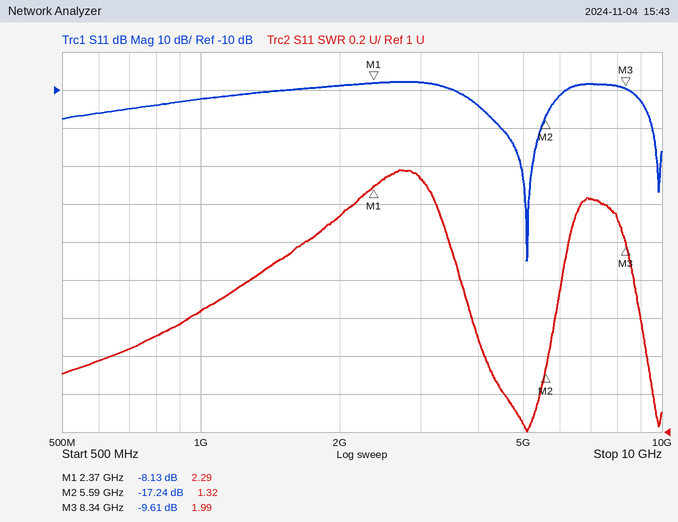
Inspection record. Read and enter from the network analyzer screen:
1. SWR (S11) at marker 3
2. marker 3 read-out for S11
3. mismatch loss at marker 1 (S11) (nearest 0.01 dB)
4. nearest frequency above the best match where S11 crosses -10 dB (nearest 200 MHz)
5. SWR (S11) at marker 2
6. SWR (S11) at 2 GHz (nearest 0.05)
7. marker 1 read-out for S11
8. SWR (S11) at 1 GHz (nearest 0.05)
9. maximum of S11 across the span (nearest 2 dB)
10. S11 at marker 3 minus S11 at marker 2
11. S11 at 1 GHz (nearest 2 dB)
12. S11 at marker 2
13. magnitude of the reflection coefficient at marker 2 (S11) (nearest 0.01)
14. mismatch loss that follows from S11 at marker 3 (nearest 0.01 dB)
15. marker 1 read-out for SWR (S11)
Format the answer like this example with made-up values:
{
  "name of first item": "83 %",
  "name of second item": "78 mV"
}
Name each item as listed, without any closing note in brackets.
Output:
{
  "SWR (S11) at marker 3": "1.99",
  "marker 3 read-out for S11": "-9.61 dB",
  "mismatch loss at marker 1 (S11)": "0.73 dB",
  "nearest frequency above the best match where S11 crosses -10 dB": "6.2 GHz",
  "SWR (S11) at marker 2": "1.32",
  "SWR (S11) at 2 GHz": "2.15",
  "marker 1 read-out for S11": "-8.13 dB",
  "SWR (S11) at 1 GHz": "1.65",
  "maximum of S11 across the span": "-8 dB",
  "S11 at marker 3 minus S11 at marker 2": "7.63 dB",
  "S11 at 1 GHz": "-12 dB",
  "S11 at marker 2": "-17.24 dB",
  "magnitude of the reflection coefficient at marker 2 (S11)": "0.14",
  "mismatch loss that follows from S11 at marker 3": "0.50 dB",
  "marker 1 read-out for SWR": "2.29"
}
